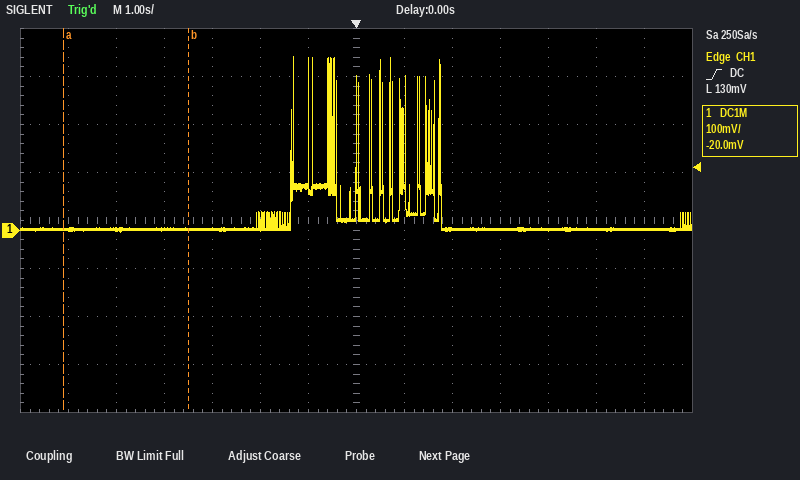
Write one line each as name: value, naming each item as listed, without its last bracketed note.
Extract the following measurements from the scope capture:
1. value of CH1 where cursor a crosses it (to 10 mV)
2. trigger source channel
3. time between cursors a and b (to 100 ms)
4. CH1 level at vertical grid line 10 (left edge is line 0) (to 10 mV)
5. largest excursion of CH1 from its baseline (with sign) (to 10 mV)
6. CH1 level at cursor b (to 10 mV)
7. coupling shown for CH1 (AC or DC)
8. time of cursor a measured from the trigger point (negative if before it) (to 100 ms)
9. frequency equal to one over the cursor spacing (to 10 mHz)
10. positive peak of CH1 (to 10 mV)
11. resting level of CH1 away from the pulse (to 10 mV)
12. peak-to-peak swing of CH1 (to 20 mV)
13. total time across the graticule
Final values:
value of CH1 where cursor a crosses it: 0 mV
trigger source channel: CH1
time between cursors a and b: 2.6 s
CH1 level at vertical grid line 10 (left edge is line 0): 0 mV
largest excursion of CH1 from its baseline (with sign): +360 mV
CH1 level at cursor b: 0 mV
coupling shown for CH1: DC
time of cursor a measured from the trigger point (negative if before it): -6.1 s
frequency equal to one over the cursor spacing: 380 mHz
positive peak of CH1: 360 mV
resting level of CH1 away from the pulse: 0 mV
peak-to-peak swing of CH1: 360 mV
total time across the graticule: 14 s
